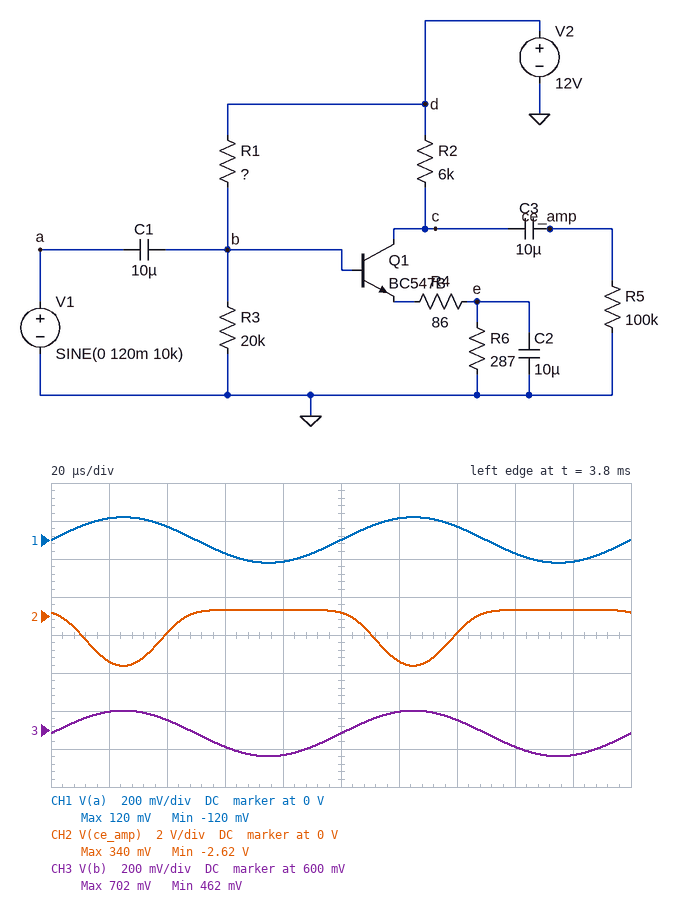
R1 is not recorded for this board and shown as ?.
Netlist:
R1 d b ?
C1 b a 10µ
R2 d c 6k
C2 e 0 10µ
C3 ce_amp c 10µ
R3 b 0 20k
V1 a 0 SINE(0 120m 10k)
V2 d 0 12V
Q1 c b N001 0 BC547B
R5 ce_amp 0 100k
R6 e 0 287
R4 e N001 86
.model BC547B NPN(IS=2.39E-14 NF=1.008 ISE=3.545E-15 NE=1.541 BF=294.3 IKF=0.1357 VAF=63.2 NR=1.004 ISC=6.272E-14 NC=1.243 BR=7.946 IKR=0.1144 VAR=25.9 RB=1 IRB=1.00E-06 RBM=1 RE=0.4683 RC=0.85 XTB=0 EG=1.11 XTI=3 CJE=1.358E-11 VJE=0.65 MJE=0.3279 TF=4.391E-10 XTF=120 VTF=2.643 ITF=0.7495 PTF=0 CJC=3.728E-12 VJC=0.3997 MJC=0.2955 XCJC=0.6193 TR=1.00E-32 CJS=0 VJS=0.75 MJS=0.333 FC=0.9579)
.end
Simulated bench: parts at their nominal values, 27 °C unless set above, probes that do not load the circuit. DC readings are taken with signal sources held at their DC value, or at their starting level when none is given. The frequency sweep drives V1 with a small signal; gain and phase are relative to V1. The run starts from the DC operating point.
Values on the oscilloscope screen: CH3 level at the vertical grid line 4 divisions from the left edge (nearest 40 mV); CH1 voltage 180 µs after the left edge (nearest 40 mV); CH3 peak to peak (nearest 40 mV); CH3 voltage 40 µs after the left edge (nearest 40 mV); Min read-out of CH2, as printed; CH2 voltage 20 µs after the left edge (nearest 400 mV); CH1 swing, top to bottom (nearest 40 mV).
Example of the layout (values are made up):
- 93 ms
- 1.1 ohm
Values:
- 480 mV
- -120 mV
- 240 mV
- 640 mV
- -2.62 V
- -2.4 V
- 240 mV
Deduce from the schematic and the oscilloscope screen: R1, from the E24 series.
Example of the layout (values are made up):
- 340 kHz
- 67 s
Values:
- 390 kΩ
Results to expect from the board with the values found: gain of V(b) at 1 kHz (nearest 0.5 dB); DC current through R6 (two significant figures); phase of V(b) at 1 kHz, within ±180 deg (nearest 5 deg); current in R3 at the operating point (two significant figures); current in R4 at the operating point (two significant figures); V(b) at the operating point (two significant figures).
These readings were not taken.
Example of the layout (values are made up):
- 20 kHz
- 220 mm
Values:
- 0 dB
- 59 µA
- 0 deg
- 29 µA
- 59 µA
- 580 mV
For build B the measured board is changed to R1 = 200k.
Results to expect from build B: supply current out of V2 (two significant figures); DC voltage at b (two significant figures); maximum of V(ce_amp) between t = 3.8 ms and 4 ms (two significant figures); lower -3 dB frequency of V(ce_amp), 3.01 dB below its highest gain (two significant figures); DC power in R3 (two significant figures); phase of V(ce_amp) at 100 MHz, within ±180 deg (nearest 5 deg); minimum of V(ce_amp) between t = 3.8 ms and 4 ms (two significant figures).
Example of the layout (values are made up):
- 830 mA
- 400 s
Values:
- 1.1 mA
- 1.0 V
- 5.0 V
- 180 Hz
- 53 µW
- 55 deg
- -5.2 V
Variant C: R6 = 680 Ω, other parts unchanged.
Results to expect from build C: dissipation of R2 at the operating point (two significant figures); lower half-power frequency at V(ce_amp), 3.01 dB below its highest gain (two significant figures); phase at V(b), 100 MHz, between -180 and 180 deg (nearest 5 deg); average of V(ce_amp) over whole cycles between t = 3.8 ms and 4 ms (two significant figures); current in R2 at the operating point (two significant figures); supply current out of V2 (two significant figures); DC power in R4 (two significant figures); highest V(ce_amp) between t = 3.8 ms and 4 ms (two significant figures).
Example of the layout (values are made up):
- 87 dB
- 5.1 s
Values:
- 10 µW
- 32 Hz
- 0 deg
- -380 mV
- 42 µA
- 71 µA
- 150 nW
- 240 mV
